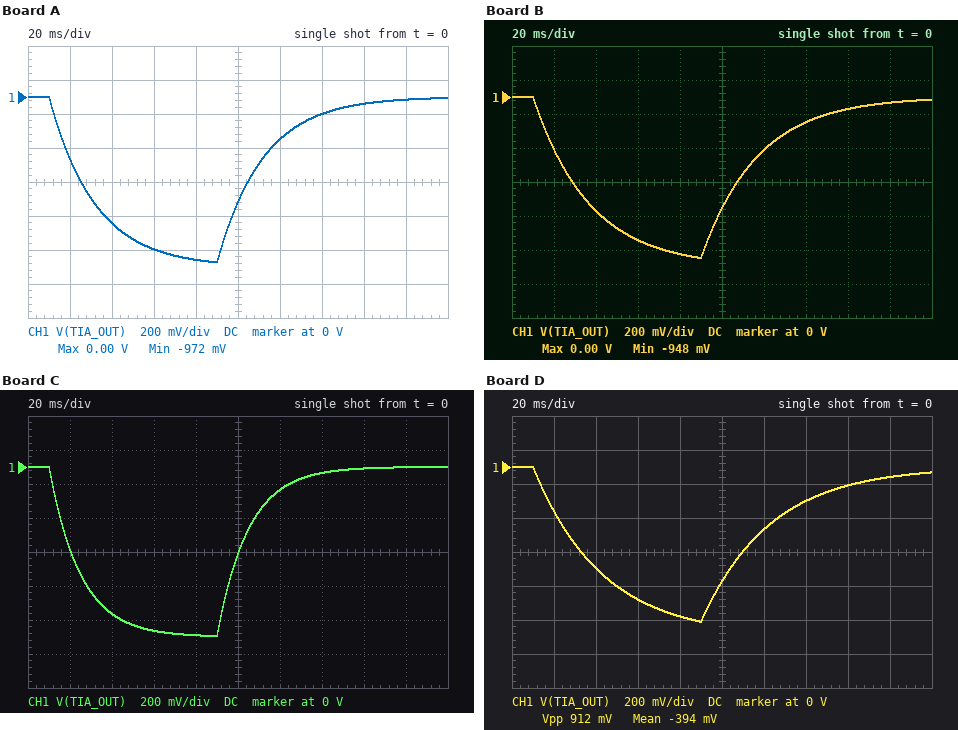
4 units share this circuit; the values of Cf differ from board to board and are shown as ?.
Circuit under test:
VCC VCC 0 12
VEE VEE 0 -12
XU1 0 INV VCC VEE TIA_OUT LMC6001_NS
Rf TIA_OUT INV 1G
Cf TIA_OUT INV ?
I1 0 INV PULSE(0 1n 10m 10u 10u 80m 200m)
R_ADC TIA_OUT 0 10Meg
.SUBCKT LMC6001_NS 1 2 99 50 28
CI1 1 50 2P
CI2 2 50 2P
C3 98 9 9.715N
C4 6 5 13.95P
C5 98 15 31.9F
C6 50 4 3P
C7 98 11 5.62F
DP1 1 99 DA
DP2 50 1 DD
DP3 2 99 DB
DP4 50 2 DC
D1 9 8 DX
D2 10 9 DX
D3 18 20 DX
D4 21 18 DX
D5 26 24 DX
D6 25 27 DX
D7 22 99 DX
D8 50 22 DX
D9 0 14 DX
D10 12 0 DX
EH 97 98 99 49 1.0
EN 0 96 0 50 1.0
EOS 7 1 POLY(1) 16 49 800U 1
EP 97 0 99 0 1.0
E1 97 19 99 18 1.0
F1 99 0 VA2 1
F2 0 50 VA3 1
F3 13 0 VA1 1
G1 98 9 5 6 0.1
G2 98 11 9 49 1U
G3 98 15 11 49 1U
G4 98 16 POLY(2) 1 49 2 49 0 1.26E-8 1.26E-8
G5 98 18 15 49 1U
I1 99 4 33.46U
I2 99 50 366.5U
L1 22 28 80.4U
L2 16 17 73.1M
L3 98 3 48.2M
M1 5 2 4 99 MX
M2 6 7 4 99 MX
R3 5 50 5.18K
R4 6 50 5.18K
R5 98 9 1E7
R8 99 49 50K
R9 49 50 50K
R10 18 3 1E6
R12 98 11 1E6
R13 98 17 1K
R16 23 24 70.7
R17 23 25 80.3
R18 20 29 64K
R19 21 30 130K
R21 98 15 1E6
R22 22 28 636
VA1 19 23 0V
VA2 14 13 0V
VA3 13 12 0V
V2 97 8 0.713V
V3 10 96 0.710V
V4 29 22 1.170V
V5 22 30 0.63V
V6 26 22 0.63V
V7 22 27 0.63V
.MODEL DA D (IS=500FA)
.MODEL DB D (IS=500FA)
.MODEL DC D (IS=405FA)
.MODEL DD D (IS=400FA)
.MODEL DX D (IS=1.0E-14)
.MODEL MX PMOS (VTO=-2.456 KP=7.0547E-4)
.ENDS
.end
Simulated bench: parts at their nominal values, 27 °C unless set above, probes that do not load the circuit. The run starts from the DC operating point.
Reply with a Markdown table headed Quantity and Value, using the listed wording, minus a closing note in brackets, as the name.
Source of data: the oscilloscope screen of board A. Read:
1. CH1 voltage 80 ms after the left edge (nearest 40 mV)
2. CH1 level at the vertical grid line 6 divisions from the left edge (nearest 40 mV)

| Quantity | Value |
|---|---|
| CH1 voltage 80 ms after the left edge | -960 mV |
| CH1 level at the vertical grid line 6 divisions from the left edge | -240 mV |
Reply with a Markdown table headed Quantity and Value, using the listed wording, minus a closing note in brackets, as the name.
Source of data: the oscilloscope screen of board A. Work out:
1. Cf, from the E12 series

| Quantity | Value |
|---|---|
| Cf, from the E12 series | 22 pF |
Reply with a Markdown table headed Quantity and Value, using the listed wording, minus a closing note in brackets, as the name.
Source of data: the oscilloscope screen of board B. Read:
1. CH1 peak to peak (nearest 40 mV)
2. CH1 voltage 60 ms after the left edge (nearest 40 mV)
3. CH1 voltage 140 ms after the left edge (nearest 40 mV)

| Quantity | Value |
|---|---|
| CH1 peak to peak | 960 mV |
| CH1 voltage 60 ms after the left edge | -840 mV |
| CH1 voltage 140 ms after the left edge | -160 mV |
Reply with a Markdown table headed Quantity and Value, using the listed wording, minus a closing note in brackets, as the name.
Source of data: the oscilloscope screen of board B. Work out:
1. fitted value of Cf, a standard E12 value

| Quantity | Value |
|---|---|
| fitted value of Cf, a standard E12 value | 27 pF |
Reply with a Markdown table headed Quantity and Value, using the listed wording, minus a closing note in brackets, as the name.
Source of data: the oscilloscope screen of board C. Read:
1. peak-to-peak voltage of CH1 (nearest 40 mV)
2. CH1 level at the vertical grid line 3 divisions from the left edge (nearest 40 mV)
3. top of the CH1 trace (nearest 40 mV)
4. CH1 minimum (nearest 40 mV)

| Quantity | Value |
|---|---|
| peak-to-peak voltage of CH1 | 1.00 V |
| CH1 level at the vertical grid line 3 divisions from the left edge | -960 mV |
| top of the CH1 trace | 0 V |
| CH1 minimum | -1.00 V |
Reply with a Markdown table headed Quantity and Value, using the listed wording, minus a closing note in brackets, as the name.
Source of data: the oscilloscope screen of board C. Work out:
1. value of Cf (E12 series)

| Quantity | Value |
|---|---|
| value of Cf | 15 pF |
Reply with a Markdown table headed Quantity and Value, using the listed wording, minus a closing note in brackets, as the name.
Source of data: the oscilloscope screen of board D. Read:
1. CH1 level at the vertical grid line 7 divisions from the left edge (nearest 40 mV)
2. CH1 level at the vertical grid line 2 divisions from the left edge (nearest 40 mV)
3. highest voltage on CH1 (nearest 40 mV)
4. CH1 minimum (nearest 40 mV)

| Quantity | Value |
|---|---|
| CH1 level at the vertical grid line 7 divisions from the left edge | -200 mV |
| CH1 level at the vertical grid line 2 divisions from the left edge | -600 mV |
| highest voltage on CH1 | 0 V |
| CH1 minimum | -920 mV |
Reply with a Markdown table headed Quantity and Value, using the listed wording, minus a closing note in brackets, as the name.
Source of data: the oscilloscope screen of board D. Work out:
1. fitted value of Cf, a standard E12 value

| Quantity | Value |
|---|---|
| fitted value of Cf, a standard E12 value | 33 pF |
